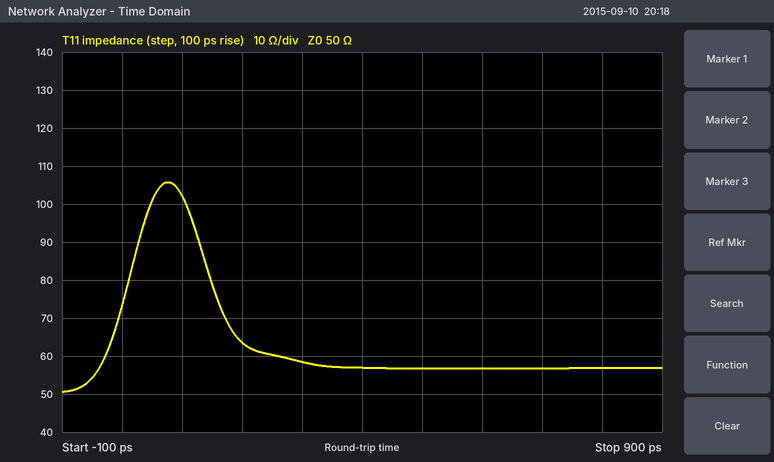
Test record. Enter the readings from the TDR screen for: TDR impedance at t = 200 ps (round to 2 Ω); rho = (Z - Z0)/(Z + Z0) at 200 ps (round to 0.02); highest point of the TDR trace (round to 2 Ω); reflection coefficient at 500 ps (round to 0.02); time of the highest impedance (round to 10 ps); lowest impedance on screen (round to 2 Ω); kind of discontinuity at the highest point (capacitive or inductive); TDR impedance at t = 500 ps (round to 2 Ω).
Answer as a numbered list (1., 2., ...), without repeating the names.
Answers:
1. 64 Ω
2. +0.12
3. 106 Ω
4. +0.06
5. 80 ps
6. 50 Ω
7. inductive
8. 56 Ω
